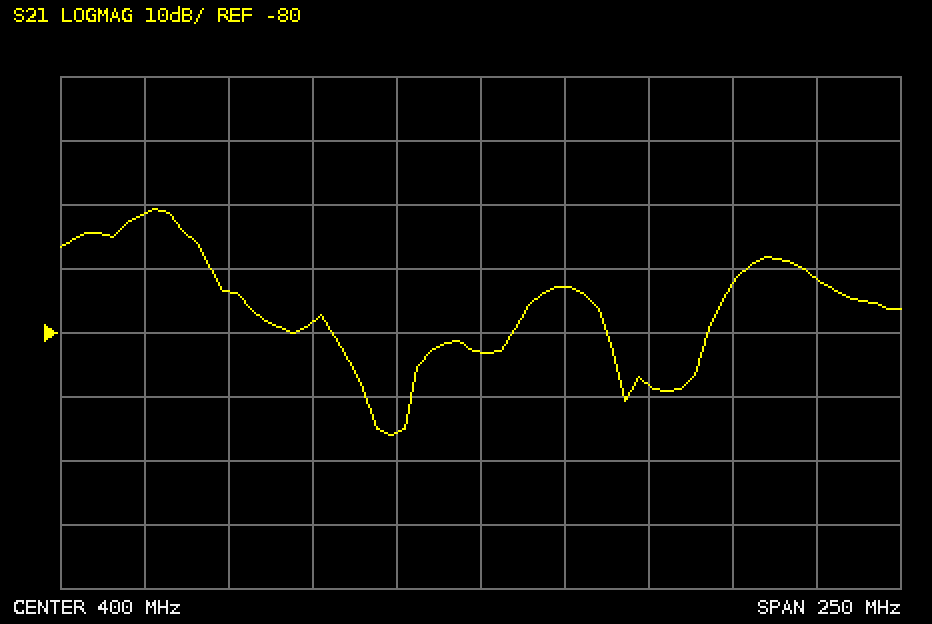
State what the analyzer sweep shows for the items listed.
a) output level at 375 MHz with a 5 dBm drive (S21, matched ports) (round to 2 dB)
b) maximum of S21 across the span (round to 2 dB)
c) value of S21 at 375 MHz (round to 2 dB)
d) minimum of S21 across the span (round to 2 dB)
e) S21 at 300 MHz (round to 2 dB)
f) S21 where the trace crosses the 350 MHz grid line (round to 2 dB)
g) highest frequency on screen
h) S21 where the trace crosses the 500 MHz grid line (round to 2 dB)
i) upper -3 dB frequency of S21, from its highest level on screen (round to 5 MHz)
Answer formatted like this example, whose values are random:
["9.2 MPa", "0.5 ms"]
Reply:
["-90 dBm", "-60 dB", "-96 dB", "-96 dB", "-62 dB", "-78 dB", "525 MHz", "-72 dB", "310 MHz"]
